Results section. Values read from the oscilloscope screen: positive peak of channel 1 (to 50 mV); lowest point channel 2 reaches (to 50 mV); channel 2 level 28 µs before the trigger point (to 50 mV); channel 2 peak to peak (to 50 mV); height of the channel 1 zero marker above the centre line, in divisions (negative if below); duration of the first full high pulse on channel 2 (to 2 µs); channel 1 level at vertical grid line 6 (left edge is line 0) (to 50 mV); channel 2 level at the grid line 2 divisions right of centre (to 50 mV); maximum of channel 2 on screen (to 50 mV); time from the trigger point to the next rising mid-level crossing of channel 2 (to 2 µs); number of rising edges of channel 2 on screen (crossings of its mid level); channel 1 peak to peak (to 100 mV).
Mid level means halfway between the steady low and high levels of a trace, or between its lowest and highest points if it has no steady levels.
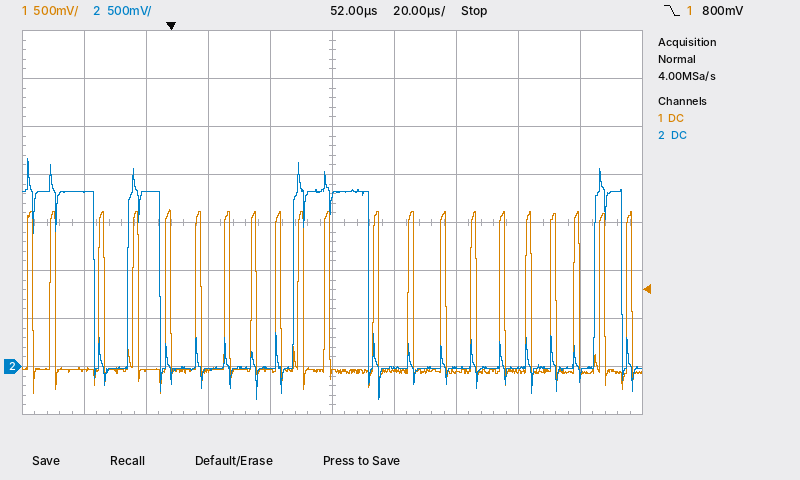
1.65 V
-350 mV
1.80 V
2.50 V
-3.0 div
10 µs
-50 mV
0 mV
2.15 V
40 µs
3
1.90 V
